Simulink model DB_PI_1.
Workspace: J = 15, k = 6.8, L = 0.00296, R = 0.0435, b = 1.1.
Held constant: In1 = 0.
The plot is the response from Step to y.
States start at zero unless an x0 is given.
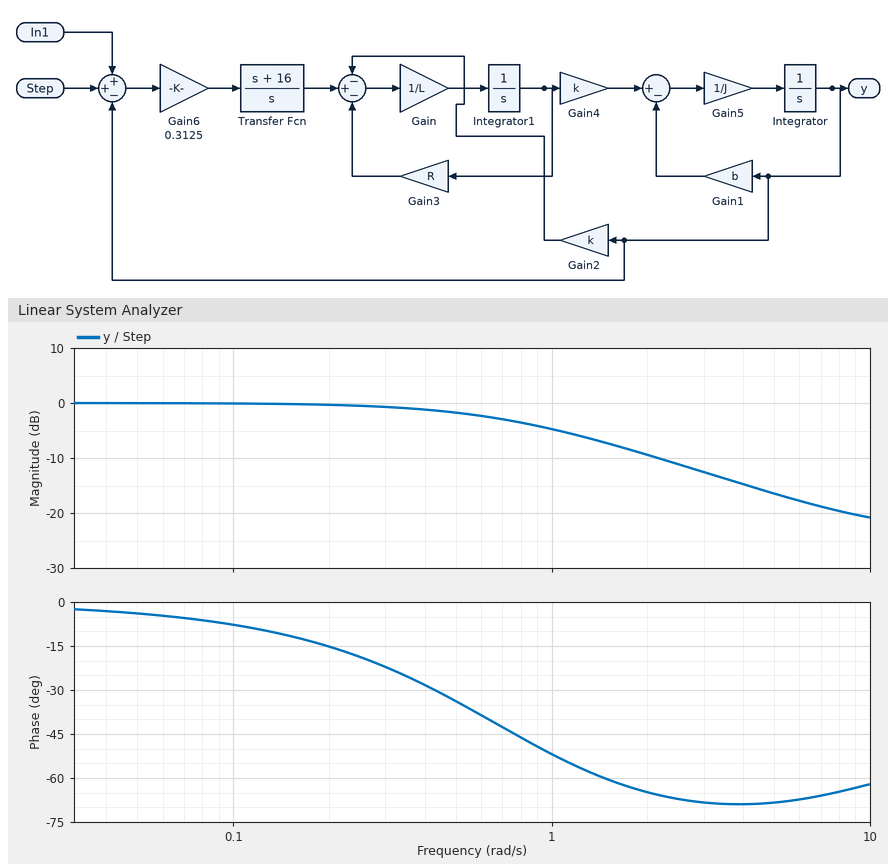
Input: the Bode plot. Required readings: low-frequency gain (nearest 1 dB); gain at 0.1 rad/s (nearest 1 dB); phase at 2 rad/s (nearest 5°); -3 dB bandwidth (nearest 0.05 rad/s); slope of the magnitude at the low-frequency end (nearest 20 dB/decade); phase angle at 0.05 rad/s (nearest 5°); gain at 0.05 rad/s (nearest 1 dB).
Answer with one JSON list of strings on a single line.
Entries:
["0 dB", "0 dB", "-65°", "0.70 rad/s", "0 dB/decade", "-5°", "0 dB"]
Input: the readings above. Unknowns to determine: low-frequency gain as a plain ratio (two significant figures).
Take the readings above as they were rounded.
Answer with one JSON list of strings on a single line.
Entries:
["1.0"]
